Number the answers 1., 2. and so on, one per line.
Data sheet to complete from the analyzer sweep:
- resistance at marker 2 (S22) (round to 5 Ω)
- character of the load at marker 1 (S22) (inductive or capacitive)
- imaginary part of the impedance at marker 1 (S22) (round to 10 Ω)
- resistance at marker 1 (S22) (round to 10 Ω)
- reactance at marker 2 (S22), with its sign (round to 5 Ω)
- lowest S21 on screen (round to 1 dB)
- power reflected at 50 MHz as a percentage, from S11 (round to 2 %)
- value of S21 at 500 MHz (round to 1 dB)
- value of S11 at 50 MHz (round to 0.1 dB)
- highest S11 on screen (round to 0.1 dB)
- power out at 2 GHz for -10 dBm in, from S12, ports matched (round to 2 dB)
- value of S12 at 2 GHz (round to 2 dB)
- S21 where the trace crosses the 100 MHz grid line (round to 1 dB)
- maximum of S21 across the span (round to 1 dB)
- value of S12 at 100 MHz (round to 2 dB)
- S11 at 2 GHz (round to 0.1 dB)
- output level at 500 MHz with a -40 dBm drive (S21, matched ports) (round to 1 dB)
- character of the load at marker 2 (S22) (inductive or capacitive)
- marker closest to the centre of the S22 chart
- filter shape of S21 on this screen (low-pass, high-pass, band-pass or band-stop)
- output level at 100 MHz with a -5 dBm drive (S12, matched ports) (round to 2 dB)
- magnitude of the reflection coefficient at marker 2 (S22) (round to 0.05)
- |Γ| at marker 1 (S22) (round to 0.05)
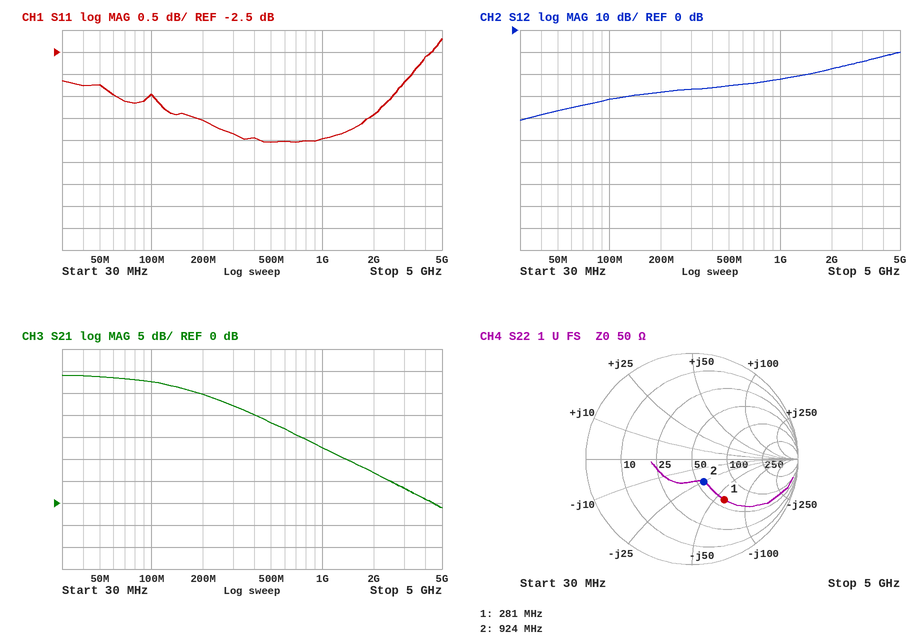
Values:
1. 55 Ω
2. capacitive
3. -60 Ω
4. 60 Ω
5. -25 Ω
6. -1 dB
7. 48 %
8. 18 dB
9. -3.2 dB
10. -2.2 dB
11. -28 dBm
12. -18 dB
13. 28 dB
14. 29 dB
15. -32 dB
16. -3.9 dB
17. -22 dBm
18. capacitive
19. marker 2
20. low-pass
21. -36 dBm
22. 0.25
23. 0.50
